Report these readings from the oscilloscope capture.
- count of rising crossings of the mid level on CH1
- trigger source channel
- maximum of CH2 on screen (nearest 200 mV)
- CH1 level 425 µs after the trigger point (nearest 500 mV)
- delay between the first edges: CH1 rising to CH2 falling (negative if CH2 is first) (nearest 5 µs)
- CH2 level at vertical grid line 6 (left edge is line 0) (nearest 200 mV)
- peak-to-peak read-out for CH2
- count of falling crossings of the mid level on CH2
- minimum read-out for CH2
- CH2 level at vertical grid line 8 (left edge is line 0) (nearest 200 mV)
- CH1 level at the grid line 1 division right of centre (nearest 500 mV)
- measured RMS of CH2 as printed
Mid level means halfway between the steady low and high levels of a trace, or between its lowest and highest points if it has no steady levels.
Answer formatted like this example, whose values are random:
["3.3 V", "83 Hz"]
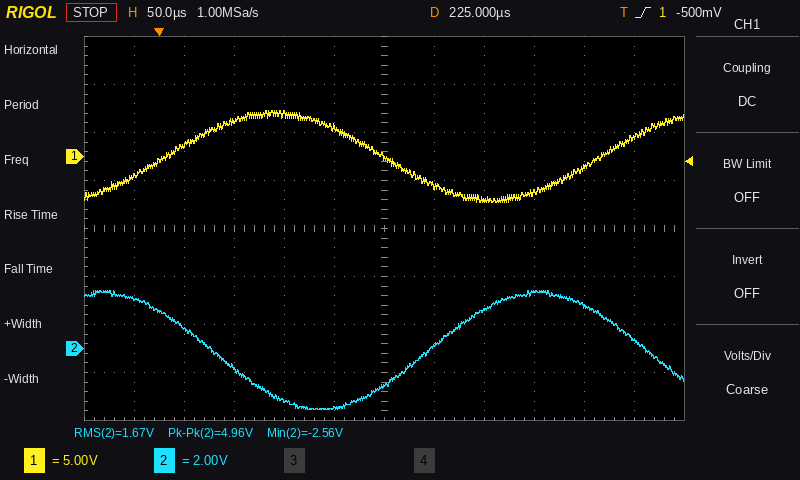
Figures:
["2", "CH1", "2.4 V", "-1.0 V", "+45 µs", "-1.6 V", "4.96 V", "2", "-2.56 V", "1.6 V", "-3.0 V", "1.67 V"]
